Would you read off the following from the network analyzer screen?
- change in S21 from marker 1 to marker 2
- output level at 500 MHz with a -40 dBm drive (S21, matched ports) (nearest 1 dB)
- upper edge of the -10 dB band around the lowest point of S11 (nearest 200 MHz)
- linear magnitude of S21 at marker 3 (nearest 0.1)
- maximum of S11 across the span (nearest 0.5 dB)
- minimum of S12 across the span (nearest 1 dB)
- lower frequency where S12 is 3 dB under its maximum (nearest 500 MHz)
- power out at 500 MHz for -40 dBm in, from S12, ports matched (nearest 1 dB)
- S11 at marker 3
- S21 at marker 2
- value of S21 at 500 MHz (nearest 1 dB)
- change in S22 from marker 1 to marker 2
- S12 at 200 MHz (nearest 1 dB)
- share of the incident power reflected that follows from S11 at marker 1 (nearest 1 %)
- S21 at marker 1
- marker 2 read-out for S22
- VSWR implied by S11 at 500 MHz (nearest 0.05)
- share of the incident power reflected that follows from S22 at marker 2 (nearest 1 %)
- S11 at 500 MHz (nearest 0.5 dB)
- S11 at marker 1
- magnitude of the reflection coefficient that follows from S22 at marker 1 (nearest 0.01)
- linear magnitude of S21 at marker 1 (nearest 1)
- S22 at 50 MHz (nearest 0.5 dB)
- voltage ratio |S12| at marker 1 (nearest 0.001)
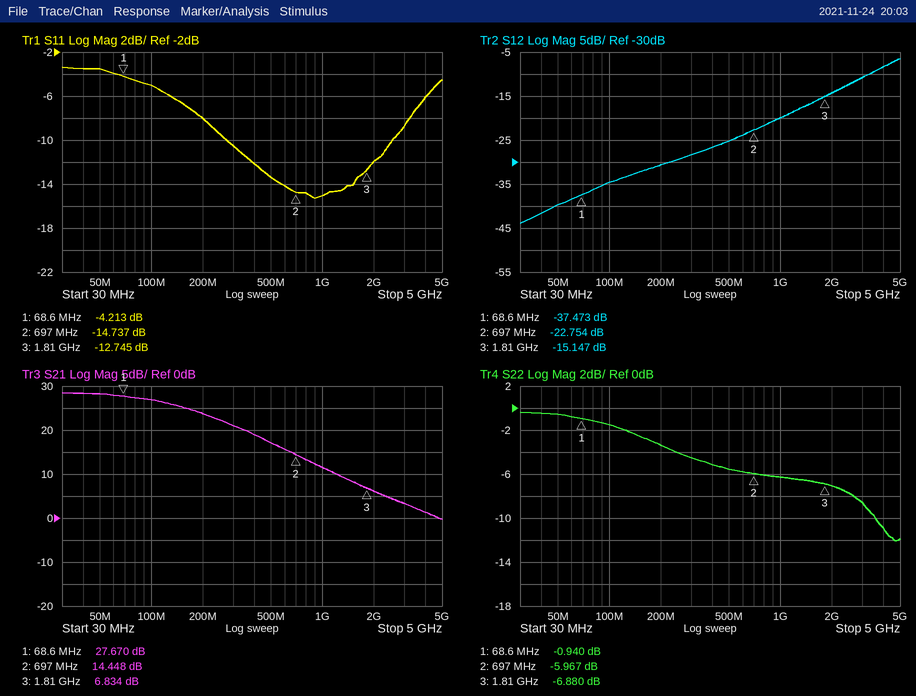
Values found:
-13.222 dB
-23 dBm
2.6 GHz
2.2
-3.5 dB
-44 dB
3.5 GHz
-65 dBm
-12.745 dB
14.448 dB
17 dB
-5.027 dB
-31 dB
38 %
27.670 dB
-5.967 dB
1.55
25 %
-13.5 dB
-4.213 dB
0.90
24
-0.5 dB
0.013
